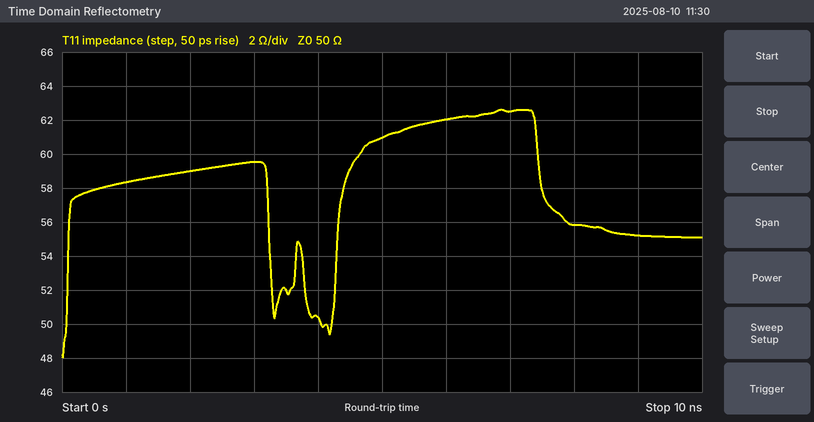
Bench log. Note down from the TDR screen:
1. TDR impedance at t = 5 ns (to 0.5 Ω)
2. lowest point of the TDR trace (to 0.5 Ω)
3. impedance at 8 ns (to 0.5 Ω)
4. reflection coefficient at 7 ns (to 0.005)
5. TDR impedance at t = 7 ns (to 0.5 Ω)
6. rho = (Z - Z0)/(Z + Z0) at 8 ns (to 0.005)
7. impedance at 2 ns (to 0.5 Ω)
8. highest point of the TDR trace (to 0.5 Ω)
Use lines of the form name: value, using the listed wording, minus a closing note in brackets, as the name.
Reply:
TDR impedance at t = 5 ns: 61.0 Ω
lowest point of the TDR trace: 48.0 Ω
impedance at 8 ns: 56.0 Ω
reflection coefficient at 7 ns: +0.110
TDR impedance at t = 7 ns: 62.5 Ω
rho = (Z - Z0)/(Z + Z0) at 8 ns: +0.055
impedance at 2 ns: 59.0 Ω
highest point of the TDR trace: 62.5 Ω
